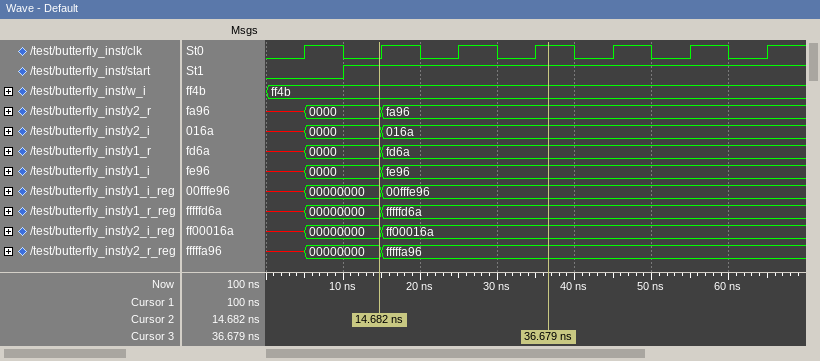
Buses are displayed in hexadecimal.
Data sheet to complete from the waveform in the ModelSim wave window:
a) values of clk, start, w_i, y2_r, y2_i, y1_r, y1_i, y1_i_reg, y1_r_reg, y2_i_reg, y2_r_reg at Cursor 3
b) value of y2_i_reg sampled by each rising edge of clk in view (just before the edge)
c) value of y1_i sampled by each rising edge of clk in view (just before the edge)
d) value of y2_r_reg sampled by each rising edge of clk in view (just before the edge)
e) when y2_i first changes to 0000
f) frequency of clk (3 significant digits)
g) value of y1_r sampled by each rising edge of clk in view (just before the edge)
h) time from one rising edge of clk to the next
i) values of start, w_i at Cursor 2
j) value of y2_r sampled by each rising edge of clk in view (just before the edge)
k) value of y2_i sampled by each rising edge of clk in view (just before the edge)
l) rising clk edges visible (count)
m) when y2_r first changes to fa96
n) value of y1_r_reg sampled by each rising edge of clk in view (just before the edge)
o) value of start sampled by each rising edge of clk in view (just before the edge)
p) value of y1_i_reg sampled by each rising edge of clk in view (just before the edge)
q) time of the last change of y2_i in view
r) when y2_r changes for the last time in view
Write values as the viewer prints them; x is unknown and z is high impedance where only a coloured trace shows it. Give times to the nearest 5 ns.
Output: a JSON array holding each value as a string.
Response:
["clk=1, start=1, w_i=ff4b, y2_r=fa96, y2_i=016a, y1_r=fd6a, y1_i=fe96, y1_i_reg=00fffe96, y1_r_reg=fffffd6a, y2_i_reg=ff00016a, y2_r_reg=fffffa96", "x, 00000000, ff00016a, ff00016a, ff00016a, ff00016a, ff00016a", "x, 0000, fe96, fe96, fe96, fe96, fe96", "x, 00000000, fffffa96, fffffa96, fffffa96, fffffa96, fffffa96", "5 ns", "100 MHz", "x, 0000, fd6a, fd6a, fd6a, fd6a, fd6a", "10 ns", "start=1, w_i=ff4b", "x, 0000, fa96, fa96, fa96, fa96, fa96", "x, 0000, 016a, 016a, 016a, 016a, 016a", "7", "15 ns", "x, 00000000, fffffd6a, fffffd6a, fffffd6a, fffffd6a, fffffd6a", "0 1 1 1 1 1 1", "x, 00000000, 00fffe96, 00fffe96, 00fffe96, 00fffe96, 00fffe96", "15 ns", "15 ns"]
